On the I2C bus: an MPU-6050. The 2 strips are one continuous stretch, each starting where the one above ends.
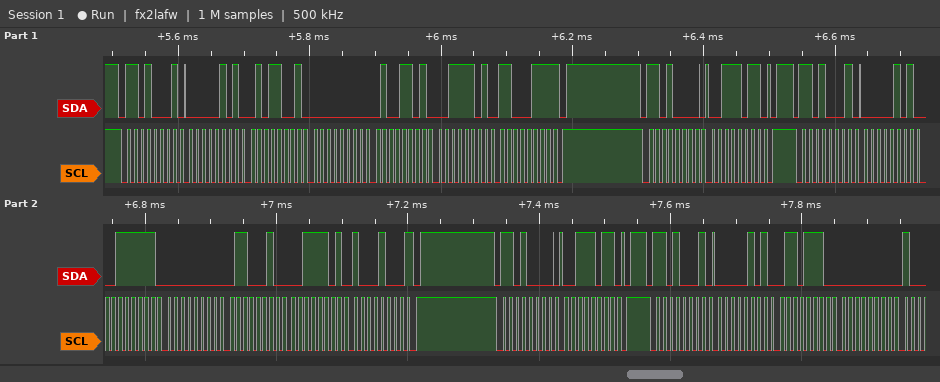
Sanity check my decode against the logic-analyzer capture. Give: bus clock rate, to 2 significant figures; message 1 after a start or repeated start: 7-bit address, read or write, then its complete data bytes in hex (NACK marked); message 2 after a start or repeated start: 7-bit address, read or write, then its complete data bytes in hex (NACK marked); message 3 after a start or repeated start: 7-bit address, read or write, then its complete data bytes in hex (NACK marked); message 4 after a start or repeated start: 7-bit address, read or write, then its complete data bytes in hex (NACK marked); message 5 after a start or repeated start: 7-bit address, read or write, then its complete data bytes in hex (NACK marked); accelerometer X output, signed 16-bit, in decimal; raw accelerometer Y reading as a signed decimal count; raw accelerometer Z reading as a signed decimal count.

100 kHz
0x68 read: 05 59 00 4D 3D C7 NACK
0x68 write: 3B
0x68 read: 05 3F 00 62 3D 88 NACK
0x68 write: 3B
0x68 read: 05 6E 00
1343
98
15752
